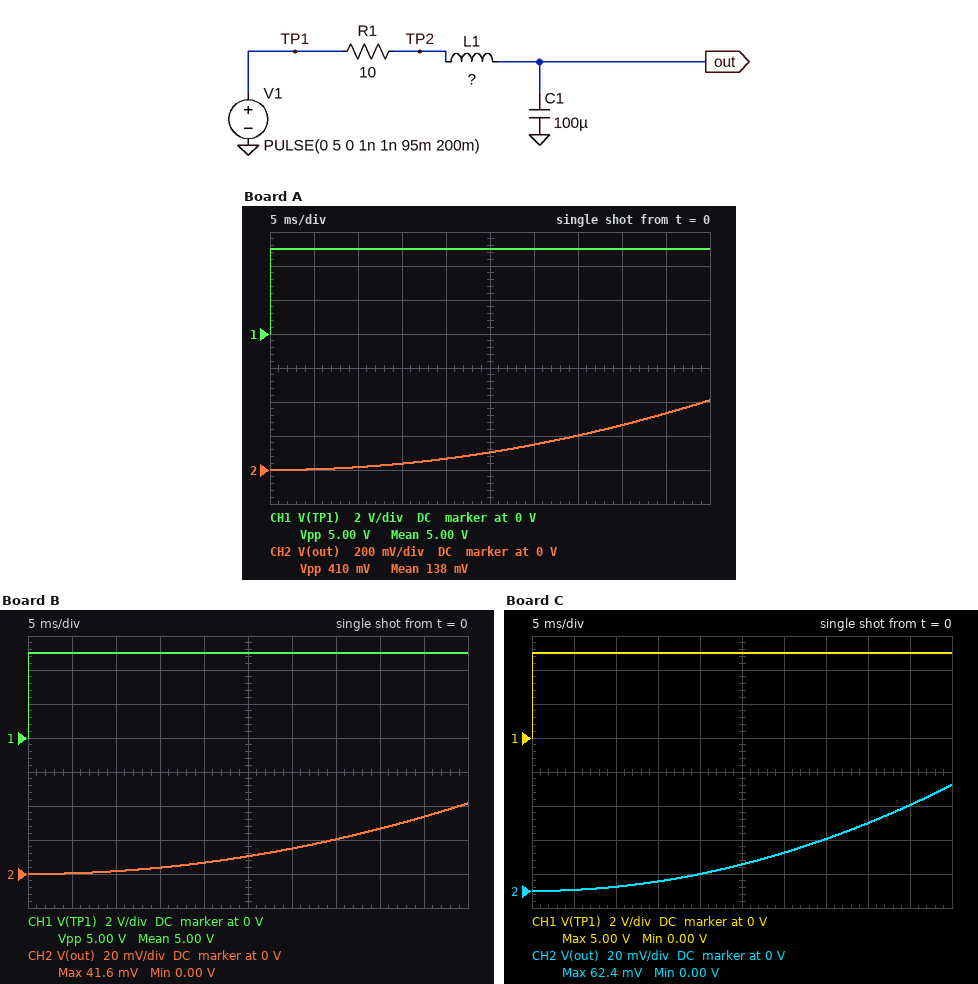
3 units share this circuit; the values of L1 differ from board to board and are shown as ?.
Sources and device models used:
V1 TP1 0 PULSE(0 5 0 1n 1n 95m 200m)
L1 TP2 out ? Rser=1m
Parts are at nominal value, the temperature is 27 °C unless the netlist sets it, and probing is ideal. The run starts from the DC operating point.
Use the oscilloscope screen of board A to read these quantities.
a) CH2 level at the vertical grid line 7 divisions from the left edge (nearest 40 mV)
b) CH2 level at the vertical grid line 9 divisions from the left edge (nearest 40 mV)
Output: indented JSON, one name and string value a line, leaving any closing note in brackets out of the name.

{
  "CH2 level at the vertical grid line 7 divisions from the left edge": "200 mV",
  "CH2 level at the vertical grid line 9 divisions from the left edge": "320 mV"
}
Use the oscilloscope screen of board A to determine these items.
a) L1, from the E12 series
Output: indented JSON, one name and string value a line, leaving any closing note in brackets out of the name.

{
  "L1, from the E12 series": "150 H"
}
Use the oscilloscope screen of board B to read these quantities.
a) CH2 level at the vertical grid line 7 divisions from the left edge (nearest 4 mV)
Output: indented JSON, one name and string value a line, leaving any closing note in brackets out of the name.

{
  "CH2 level at the vertical grid line 7 divisions from the left edge": "20 mV"
}
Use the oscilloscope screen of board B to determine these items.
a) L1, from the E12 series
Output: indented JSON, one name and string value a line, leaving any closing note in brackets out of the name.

{
  "L1, from the E12 series": "1.5 kH"
}
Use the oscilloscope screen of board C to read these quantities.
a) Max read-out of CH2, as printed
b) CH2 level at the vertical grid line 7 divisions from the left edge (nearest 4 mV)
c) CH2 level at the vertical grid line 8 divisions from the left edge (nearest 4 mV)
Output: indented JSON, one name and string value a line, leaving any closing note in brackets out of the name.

{
  "Max read-out of CH2, as printed": "62.4 mV",
  "CH2 level at the vertical grid line 7 divisions from the left edge": "32 mV",
  "CH2 level at the vertical grid line 8 divisions from the left edge": "40 mV"
}
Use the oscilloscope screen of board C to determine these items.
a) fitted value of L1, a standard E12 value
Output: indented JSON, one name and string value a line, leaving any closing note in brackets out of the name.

{
  "fitted value of L1, a standard E12 value": "1 kH"
}
